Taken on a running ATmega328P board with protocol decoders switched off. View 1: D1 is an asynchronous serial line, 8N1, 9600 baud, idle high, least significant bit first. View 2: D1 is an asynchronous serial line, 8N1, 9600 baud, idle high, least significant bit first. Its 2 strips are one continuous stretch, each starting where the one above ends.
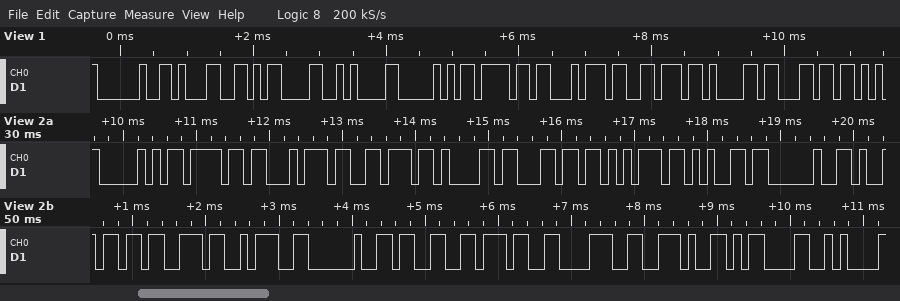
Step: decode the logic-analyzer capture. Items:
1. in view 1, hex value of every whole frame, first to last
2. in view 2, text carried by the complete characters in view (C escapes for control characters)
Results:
20 31 0D 0A 50 6F 74 76 61 6C
"Potvalue is: 378.\r\n"
